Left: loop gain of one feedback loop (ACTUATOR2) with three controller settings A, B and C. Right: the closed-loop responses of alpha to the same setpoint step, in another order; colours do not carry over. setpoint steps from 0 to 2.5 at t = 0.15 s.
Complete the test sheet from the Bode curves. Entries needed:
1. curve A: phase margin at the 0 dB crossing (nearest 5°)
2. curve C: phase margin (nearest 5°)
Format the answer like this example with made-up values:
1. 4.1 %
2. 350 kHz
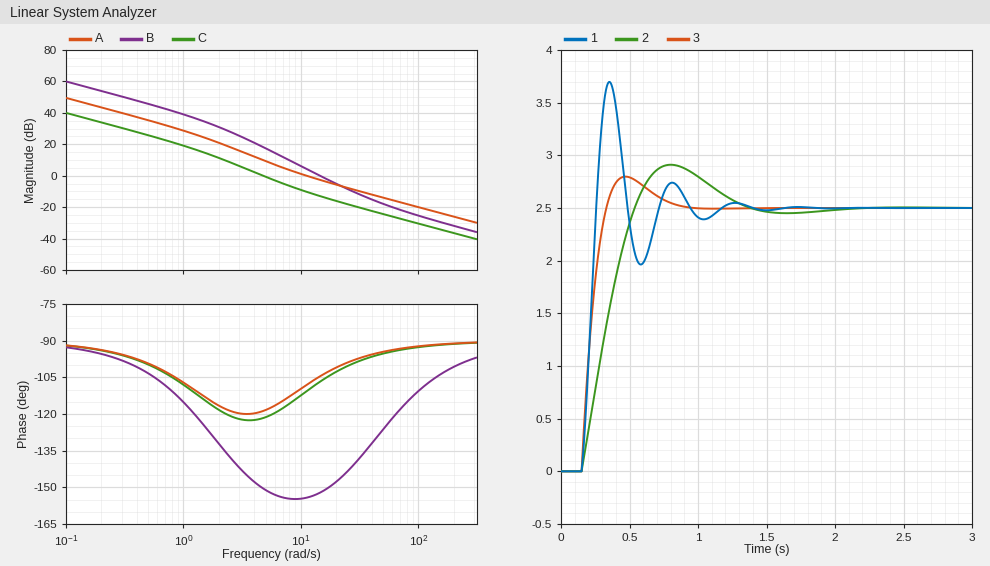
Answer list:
1. 70°
2. 60°
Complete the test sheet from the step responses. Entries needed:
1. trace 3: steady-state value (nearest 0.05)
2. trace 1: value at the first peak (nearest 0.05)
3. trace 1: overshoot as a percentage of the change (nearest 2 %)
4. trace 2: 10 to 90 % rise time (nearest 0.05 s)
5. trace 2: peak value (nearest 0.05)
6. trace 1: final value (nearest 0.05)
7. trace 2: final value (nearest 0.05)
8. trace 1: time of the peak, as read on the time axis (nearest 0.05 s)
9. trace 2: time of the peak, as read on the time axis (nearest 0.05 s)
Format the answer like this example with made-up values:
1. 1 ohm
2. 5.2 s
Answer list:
1. 2.50
2. 3.70
3. 48 %
4. 0.30 s
5. 2.90
6. 2.50
7. 2.50
8. 0.35 s
9. 0.80 s
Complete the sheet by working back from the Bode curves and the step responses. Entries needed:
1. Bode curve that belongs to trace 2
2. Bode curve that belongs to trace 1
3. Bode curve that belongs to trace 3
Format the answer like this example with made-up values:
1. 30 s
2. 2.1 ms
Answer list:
1. C
2. B
3. A
